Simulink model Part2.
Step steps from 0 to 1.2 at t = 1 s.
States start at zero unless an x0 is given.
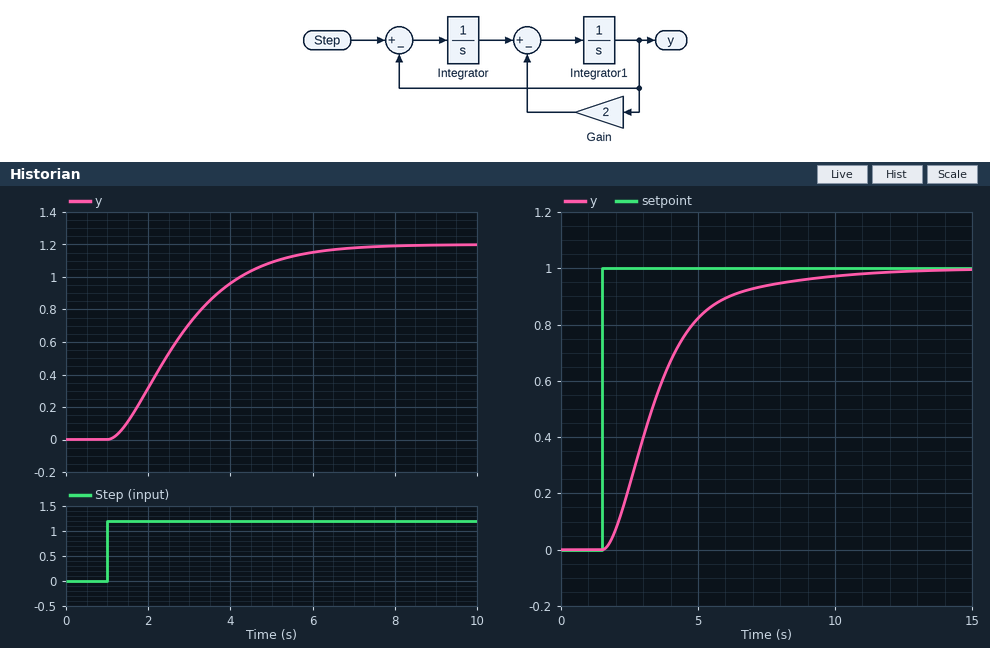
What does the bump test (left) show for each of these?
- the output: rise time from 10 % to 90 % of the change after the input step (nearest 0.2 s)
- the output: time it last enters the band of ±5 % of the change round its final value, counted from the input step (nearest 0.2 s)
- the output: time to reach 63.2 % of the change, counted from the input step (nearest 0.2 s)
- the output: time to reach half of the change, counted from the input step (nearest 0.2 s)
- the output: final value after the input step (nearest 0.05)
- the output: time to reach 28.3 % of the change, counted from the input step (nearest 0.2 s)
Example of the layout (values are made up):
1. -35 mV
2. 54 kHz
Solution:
1. 3.4 s
2. 4.8 s
3. 2.2 s
4. 1.6 s
5. 1.20
6. 1.0 s
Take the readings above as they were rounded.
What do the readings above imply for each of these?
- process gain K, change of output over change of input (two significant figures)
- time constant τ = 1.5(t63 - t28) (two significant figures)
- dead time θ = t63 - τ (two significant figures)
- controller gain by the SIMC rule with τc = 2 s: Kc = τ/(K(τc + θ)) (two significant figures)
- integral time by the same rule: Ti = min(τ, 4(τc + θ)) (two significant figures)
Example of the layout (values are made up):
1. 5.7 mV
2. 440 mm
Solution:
1. 1.0
2. 1.8 s
3. 0.40 s
4. 0.75
5. 1.8 s
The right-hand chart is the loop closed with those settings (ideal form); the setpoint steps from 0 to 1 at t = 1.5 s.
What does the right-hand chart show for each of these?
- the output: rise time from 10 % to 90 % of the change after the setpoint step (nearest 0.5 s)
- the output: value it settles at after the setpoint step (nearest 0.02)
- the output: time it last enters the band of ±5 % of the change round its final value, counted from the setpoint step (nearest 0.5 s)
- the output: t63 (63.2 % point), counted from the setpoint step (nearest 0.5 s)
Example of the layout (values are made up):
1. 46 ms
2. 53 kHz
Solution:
1. 4.0 s
2. 1.00
3. 6.5 s
4. 2.5 s
